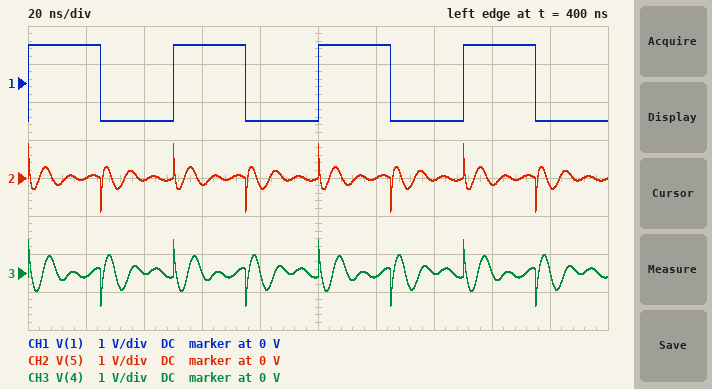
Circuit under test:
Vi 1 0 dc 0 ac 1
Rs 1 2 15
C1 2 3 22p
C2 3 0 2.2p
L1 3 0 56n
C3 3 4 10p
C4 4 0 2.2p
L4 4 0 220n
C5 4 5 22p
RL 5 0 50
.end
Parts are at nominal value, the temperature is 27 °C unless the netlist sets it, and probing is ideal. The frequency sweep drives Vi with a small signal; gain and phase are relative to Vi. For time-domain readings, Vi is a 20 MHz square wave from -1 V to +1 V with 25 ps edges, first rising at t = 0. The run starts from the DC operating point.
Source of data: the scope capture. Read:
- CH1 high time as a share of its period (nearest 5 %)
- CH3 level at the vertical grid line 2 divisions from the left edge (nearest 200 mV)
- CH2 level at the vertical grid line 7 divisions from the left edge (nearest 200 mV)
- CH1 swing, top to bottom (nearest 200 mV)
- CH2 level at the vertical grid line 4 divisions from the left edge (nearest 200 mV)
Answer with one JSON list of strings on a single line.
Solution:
["50 %", "0 V", "0 V", "2.0 V", "-200 mV"]
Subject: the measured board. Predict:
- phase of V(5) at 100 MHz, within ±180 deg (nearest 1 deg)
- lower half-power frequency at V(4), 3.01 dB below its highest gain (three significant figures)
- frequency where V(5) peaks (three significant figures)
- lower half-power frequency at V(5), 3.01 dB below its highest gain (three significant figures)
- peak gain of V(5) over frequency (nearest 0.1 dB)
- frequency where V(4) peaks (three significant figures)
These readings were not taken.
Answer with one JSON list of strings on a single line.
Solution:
["-127 deg", "109 MHz", "125 MHz", "111 MHz", "-1.4 dB", "124 MHz"]
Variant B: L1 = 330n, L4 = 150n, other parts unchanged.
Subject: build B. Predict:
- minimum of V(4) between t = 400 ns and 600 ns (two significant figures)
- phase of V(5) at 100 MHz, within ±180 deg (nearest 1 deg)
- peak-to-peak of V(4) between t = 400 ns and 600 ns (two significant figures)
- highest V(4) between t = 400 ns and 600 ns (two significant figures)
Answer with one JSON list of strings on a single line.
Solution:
["-1.0 V", "113 deg", "2.0 V", "1.0 V"]
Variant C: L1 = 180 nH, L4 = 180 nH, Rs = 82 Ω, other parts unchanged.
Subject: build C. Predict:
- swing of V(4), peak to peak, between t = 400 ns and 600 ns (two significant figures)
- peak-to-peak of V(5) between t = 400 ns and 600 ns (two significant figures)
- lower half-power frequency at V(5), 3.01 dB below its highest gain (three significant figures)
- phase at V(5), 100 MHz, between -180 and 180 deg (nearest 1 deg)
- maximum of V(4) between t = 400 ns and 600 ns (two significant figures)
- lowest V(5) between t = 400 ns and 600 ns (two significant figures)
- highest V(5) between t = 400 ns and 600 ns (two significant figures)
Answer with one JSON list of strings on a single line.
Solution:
["1.1 V", "660 mV", "56.7 MHz", "123 deg", "530 mV", "-330 mV", "330 mV"]
